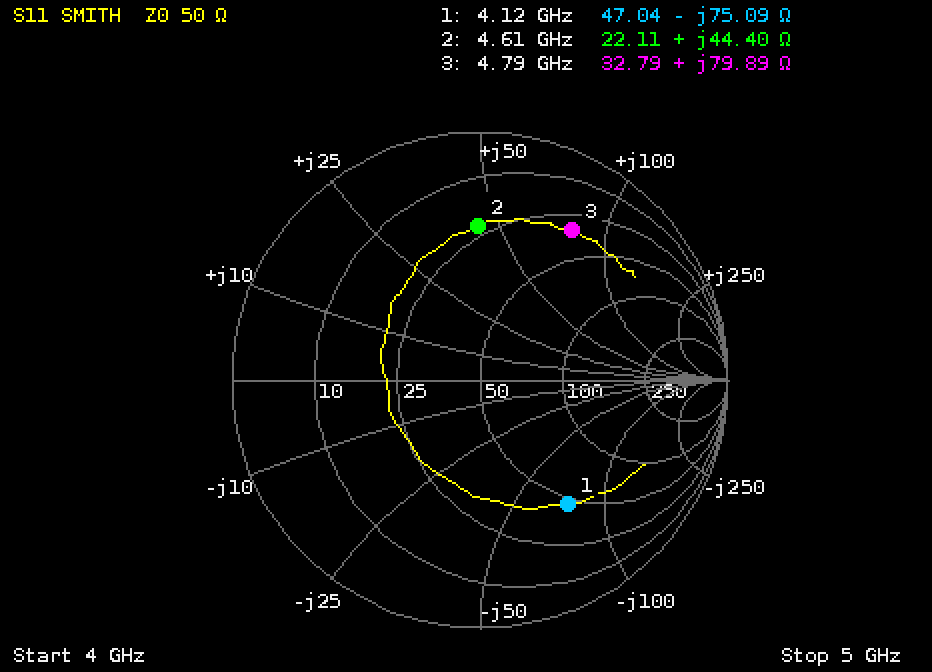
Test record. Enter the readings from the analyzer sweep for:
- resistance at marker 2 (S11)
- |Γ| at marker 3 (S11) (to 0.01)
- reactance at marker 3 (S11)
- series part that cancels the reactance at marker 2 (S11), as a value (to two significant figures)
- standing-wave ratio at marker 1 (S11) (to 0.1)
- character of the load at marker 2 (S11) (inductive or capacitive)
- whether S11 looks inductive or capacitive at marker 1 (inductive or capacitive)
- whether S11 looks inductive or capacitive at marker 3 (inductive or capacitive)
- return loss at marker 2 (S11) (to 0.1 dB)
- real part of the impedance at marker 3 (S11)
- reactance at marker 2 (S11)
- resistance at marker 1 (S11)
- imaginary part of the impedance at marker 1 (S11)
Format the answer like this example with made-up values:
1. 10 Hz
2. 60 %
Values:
1. 22.11 Ω
2. 0.71
3. +79.89 Ω
4. 780 fF
5. 4.2
6. inductive
7. capacitive
8. inductive
9. 4.2 dB
10. 32.79 Ω
11. +44.40 Ω
12. 47.04 Ω
13. -75.09 Ω
